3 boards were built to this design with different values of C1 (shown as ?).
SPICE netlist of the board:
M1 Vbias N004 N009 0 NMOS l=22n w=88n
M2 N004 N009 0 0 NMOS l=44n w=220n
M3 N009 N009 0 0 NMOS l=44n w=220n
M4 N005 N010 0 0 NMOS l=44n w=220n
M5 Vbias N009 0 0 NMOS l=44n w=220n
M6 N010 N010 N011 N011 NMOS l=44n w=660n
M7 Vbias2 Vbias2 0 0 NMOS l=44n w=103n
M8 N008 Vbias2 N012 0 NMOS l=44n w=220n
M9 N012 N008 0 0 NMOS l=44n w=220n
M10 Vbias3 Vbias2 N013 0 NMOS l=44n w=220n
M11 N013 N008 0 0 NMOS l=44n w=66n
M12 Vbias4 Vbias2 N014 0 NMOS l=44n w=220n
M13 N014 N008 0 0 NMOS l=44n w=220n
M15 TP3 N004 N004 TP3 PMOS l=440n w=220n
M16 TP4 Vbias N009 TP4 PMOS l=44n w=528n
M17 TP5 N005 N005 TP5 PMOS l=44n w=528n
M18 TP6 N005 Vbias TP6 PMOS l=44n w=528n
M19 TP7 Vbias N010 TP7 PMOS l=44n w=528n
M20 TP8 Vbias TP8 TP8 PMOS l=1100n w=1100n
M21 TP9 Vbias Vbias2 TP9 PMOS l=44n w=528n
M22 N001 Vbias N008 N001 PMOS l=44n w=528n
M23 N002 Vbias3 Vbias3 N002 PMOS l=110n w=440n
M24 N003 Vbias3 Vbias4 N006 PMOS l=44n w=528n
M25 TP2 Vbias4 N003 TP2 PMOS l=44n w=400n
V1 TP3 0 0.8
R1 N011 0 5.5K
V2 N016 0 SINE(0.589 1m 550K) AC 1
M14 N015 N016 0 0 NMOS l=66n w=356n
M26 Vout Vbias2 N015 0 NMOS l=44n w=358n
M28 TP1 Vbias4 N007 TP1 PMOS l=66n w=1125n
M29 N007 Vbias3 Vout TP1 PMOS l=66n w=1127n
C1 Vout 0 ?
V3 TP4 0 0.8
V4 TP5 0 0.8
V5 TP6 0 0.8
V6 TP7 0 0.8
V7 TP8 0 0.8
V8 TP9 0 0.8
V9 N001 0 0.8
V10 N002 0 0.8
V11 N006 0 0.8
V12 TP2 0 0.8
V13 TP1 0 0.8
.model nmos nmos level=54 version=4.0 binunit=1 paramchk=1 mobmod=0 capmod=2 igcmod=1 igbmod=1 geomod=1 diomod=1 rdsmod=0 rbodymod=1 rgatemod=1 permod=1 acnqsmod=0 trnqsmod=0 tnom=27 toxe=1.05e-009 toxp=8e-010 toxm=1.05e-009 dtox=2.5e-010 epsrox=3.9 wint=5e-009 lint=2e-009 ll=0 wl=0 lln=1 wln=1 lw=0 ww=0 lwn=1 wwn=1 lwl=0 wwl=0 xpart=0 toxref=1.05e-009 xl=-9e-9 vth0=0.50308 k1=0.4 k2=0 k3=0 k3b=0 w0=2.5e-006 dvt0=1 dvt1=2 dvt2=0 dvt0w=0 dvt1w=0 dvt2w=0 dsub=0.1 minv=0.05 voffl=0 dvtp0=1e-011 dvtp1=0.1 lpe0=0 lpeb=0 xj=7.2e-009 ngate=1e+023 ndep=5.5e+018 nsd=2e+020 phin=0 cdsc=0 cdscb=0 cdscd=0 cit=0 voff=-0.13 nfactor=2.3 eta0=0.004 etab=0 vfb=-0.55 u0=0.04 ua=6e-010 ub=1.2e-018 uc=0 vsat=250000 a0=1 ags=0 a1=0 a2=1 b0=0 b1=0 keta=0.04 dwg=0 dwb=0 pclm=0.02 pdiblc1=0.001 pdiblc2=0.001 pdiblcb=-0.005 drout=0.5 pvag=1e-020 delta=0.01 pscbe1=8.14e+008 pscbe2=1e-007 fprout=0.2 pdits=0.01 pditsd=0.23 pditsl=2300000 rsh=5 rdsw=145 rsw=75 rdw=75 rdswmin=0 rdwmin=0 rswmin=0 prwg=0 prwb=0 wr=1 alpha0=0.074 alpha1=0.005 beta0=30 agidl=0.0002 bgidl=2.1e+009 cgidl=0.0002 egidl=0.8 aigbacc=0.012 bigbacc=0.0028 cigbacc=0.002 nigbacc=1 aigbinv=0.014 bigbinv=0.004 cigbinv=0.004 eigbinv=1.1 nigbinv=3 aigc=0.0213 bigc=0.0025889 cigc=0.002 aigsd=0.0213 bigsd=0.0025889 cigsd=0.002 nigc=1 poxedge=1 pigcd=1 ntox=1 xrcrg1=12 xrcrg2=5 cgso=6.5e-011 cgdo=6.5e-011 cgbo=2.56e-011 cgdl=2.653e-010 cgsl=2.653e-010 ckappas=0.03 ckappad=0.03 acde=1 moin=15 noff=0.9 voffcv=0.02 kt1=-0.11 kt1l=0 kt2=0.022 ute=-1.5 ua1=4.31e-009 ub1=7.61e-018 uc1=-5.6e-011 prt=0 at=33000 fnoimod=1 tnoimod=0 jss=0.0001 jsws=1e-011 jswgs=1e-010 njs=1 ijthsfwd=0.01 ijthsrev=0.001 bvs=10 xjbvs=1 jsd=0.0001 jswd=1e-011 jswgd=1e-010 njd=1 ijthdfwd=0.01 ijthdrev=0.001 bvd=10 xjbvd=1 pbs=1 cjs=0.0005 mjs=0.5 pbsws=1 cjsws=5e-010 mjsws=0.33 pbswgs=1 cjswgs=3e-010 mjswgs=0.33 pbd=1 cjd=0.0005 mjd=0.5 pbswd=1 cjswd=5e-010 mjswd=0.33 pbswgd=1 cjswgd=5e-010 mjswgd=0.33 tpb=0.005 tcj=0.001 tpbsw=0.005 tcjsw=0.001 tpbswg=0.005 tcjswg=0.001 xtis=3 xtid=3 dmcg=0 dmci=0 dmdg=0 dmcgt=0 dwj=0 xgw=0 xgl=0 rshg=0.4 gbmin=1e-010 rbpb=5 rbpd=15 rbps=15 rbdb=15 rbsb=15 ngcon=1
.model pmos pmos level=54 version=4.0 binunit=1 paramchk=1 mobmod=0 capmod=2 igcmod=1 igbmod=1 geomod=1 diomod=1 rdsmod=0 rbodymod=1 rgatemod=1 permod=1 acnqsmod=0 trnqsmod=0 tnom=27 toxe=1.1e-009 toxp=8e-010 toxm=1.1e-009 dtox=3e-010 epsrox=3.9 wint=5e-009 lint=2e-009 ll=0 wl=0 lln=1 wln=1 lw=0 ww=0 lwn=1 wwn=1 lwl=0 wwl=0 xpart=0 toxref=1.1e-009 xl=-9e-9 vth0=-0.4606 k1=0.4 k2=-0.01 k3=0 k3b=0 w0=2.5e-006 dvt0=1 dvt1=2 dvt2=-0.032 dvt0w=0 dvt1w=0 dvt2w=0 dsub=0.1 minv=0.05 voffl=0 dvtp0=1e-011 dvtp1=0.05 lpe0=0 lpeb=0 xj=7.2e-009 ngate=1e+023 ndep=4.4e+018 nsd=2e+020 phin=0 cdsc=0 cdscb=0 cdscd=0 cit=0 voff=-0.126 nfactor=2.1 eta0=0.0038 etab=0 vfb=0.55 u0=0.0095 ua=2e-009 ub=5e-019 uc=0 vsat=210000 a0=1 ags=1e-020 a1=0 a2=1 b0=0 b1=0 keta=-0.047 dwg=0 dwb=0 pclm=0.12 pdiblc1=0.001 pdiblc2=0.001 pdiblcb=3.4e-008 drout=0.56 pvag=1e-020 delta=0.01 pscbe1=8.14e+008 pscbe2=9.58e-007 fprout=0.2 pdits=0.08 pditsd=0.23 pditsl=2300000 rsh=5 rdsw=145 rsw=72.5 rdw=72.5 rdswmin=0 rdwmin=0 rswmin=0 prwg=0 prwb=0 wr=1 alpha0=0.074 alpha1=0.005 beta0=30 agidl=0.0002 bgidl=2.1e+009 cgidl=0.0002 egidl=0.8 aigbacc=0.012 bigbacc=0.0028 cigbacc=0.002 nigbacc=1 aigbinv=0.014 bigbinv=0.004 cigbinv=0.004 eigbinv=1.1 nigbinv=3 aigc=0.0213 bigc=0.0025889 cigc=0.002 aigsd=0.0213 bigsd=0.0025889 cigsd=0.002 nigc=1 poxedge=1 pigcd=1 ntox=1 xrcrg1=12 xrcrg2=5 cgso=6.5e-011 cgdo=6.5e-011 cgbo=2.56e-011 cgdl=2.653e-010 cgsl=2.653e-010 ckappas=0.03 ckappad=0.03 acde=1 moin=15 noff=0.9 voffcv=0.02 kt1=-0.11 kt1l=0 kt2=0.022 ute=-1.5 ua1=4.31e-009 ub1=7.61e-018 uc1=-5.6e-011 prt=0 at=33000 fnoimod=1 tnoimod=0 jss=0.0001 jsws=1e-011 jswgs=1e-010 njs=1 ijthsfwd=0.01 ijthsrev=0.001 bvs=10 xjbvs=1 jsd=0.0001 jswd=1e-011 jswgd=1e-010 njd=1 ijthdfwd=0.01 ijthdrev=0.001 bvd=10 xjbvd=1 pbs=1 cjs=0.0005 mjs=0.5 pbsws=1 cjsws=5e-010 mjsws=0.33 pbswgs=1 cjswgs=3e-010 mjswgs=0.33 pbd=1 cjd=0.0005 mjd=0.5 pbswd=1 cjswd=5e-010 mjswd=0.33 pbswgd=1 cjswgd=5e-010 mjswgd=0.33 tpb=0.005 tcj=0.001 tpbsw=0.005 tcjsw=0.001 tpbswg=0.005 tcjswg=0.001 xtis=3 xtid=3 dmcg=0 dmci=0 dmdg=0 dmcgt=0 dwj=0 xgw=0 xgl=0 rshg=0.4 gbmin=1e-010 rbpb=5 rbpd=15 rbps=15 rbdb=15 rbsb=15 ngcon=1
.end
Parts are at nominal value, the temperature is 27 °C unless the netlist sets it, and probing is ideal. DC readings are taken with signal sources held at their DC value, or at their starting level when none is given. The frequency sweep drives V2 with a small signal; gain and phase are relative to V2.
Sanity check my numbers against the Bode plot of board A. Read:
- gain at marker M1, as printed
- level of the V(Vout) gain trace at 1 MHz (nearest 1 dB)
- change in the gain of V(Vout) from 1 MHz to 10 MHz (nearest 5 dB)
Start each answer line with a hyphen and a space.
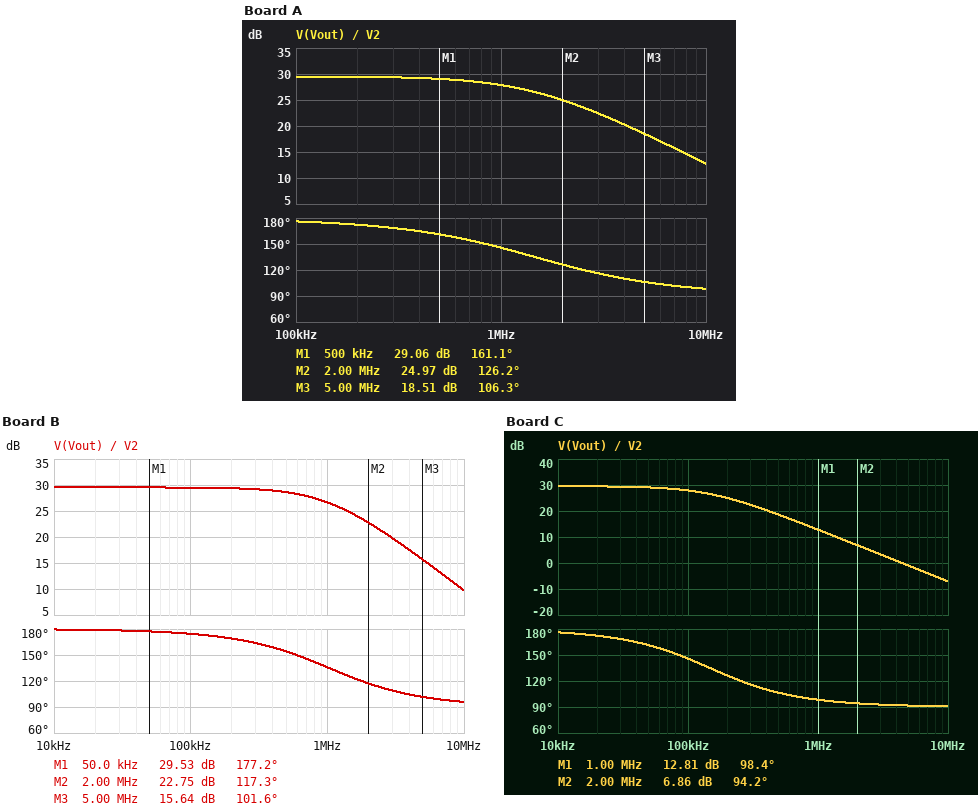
- 29.06 dB
- 28 dB
- -15 dB
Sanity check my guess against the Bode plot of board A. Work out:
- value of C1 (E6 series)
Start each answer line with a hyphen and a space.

- 330 fF
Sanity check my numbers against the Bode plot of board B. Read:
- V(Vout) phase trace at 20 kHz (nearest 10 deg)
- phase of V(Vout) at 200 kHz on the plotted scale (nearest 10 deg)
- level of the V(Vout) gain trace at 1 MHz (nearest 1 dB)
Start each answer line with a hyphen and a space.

- 180 deg
- 170 deg
- 27 dB
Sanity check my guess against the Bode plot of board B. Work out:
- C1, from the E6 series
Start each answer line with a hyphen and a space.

- 470 fF
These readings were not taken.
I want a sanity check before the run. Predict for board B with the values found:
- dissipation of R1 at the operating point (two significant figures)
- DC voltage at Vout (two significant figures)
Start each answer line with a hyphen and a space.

- 830 nW
- 460 mV
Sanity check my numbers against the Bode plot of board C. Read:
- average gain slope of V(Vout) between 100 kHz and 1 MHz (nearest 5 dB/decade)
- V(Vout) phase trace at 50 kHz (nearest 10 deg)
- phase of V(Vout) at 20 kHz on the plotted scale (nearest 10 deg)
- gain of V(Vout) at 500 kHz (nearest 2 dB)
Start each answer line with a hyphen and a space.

- -15 dB/decade
- 160 deg
- 170 deg
- 18 dB
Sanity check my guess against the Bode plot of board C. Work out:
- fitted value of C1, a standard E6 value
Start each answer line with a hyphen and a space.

- 3.3 pF
